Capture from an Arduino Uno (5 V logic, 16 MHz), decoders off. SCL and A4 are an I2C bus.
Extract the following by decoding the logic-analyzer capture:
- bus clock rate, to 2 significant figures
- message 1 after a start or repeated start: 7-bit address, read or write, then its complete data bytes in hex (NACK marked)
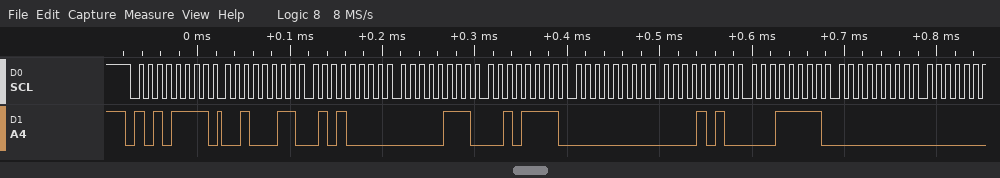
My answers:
100 kHz
0x57 read: 23 50 07 2F 00 0A 1F 00
